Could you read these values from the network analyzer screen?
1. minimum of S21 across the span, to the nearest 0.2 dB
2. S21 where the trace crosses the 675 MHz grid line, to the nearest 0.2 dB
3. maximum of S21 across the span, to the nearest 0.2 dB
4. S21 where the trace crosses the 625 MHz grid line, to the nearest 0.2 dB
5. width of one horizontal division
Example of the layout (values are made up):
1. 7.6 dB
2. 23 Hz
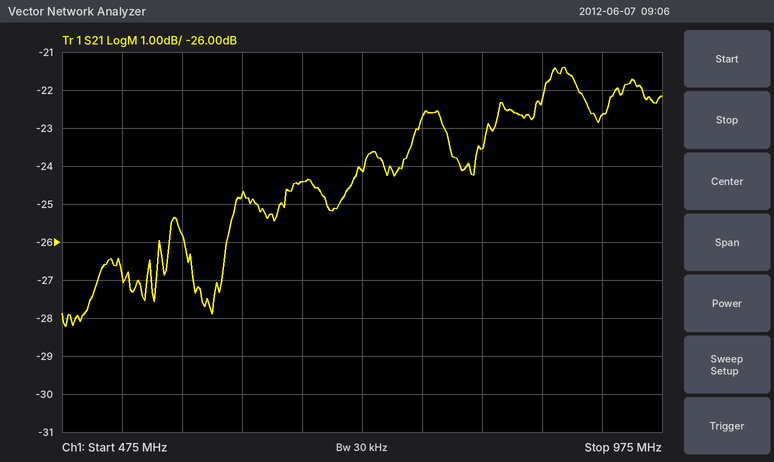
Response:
1. -28.2 dB
2. -24.4 dB
3. -21.4 dB
4. -24.8 dB
5. 50 MHz
